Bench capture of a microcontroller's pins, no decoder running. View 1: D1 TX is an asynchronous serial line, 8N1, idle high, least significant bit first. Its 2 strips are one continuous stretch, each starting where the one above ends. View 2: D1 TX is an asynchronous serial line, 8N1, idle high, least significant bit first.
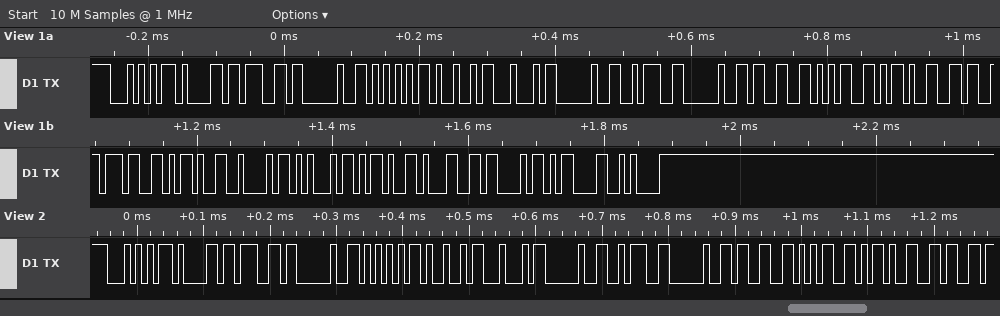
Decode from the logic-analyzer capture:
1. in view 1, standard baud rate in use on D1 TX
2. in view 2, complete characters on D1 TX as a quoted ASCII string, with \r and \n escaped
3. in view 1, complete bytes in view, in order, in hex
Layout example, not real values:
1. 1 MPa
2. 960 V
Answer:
1. 115200 baud
2. "Tag UID : 35-6"
3. 54 61 67 20 55 49 44 20 3A 20 33 35 2D 36 37 2D 42 45 2D 31 43 0D 0A
